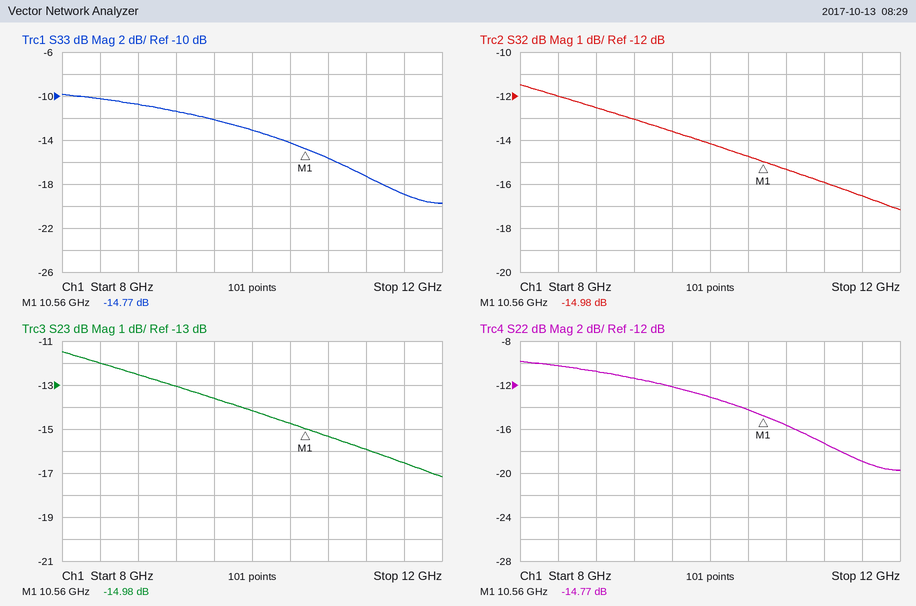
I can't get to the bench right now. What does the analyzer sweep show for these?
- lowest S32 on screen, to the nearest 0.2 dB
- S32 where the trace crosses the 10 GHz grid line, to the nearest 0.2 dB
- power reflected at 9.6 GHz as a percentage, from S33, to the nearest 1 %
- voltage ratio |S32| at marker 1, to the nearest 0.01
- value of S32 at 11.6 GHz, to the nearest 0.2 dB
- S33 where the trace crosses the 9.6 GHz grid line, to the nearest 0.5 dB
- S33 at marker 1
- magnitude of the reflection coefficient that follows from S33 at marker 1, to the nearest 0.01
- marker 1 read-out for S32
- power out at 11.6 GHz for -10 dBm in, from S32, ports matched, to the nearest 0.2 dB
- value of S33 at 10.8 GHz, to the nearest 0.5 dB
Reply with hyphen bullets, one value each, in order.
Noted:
- -17.2 dB
- -14.2 dB
- 6 %
- 0.18
- -16.6 dB
- -12.0 dB
- -14.77 dB
- 0.18
- -14.98 dB
- -26.6 dBm
- -15.5 dB
